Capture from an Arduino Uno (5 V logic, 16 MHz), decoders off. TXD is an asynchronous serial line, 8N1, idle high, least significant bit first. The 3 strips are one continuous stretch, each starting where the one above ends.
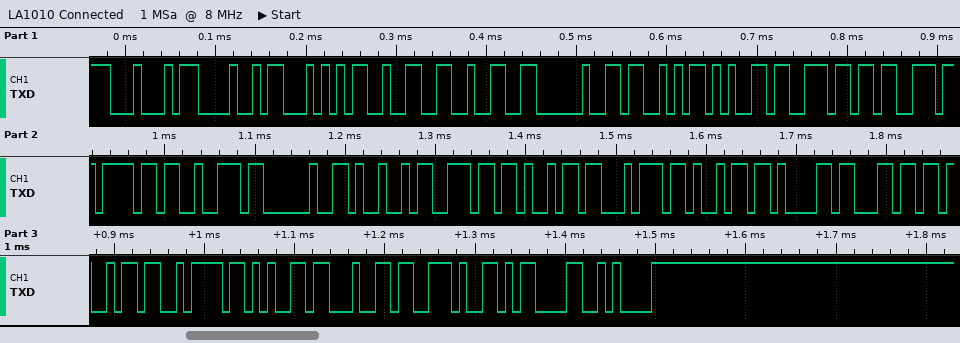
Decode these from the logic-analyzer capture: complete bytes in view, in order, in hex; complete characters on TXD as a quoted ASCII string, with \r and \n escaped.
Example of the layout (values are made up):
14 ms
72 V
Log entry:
44 48 54 32 32 20 53 65 6E 73 6F 72 20 49 6E 69 74 69 61 6C 69 7A 65 64 2E 0D 0A
"DHT22 Sensor Initialized.\r\n"
